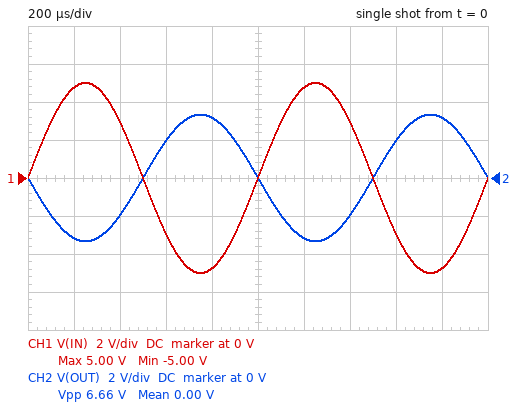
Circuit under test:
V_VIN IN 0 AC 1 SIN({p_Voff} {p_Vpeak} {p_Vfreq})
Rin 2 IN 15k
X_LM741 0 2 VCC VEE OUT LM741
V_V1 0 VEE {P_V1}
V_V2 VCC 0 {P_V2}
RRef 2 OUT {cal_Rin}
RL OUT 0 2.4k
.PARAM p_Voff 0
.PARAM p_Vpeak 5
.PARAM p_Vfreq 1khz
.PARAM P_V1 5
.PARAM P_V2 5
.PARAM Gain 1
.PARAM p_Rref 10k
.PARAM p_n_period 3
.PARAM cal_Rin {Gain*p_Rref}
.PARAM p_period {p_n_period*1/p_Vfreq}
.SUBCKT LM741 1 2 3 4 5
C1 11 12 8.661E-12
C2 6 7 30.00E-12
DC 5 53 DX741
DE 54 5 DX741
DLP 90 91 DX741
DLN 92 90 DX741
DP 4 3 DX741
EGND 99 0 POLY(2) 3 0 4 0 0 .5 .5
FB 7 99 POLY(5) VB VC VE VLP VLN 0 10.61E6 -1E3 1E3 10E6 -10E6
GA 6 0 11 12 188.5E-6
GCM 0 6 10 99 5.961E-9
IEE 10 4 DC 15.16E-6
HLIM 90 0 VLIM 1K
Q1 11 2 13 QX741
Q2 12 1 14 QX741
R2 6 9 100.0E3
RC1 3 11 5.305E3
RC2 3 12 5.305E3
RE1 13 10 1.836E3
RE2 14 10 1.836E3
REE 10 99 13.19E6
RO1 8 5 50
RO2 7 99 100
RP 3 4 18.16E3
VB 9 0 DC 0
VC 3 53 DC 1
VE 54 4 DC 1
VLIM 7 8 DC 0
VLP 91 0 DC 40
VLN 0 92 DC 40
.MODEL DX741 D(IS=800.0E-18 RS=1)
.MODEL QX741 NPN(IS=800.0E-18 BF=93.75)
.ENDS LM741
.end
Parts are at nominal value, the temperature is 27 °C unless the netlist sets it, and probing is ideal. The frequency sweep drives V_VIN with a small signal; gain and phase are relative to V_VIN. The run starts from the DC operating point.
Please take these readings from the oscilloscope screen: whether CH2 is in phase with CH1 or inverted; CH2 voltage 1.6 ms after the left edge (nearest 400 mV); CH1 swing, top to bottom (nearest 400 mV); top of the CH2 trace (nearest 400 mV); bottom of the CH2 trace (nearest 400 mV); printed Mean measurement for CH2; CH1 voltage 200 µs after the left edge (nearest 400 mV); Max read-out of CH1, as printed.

inverted
2.0 V
10.0 V
3.2 V
-3.2 V
0.00 V
4.8 V
5.00 V
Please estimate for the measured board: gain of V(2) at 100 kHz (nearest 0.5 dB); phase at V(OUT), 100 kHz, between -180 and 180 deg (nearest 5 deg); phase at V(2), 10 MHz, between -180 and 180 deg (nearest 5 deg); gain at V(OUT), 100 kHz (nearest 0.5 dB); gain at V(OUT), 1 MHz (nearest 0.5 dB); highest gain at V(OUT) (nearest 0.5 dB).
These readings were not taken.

-23.5 dB
170 deg
0 deg
-3.5 dB
-8.0 dB
-3.5 dB
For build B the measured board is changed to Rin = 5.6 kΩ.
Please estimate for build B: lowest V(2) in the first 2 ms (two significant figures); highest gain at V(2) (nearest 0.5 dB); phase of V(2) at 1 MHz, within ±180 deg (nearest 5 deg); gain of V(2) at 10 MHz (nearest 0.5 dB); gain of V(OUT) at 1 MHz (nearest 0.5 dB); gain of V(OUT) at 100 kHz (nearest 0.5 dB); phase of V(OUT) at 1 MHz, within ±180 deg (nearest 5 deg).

-1.5 V
-3.0 dB
15 deg
-4.0 dB
-4.5 dB
5.0 dB
75 deg
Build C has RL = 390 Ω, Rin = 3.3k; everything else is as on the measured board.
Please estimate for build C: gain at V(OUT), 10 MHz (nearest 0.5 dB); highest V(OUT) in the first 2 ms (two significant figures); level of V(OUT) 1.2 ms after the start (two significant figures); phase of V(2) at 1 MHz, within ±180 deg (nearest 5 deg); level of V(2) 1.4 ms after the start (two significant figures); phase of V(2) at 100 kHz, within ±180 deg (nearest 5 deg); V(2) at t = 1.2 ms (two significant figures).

-36.5 dB
4.8 V
-4.8 V
10 deg
1.0 V
70 deg
2.4 V
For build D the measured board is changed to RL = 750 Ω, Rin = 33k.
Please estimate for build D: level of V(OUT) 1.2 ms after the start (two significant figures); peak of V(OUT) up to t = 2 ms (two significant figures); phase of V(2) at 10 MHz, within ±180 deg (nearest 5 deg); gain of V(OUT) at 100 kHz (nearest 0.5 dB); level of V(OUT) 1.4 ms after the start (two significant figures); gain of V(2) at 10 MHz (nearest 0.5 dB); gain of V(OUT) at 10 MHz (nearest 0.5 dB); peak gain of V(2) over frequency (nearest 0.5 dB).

-1.4 V
1.5 V
0 deg
-10.5 dB
-890 mV
-12.5 dB
-46.5 dB
-11.0 dB
